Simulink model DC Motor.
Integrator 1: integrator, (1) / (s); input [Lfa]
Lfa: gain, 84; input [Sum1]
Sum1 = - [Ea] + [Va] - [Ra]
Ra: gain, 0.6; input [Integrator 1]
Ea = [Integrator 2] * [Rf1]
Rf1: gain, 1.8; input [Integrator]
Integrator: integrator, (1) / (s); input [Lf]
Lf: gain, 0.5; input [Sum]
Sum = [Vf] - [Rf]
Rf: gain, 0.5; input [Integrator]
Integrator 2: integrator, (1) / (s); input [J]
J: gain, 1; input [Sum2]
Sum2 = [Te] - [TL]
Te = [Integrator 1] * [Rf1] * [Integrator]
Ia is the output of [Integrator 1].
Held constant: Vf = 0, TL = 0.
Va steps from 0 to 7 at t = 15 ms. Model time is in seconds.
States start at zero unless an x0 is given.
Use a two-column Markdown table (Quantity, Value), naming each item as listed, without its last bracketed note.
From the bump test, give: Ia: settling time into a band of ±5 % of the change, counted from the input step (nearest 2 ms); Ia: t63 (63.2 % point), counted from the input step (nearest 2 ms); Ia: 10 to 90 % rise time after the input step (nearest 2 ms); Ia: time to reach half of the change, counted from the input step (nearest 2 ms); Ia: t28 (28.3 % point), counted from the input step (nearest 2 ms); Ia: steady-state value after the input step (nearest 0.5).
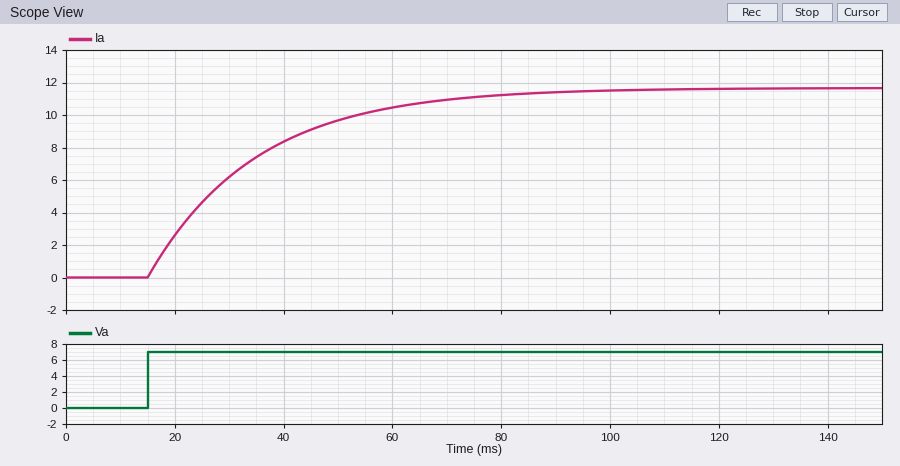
| Quantity | Value |
|---|---|
| Ia: settling time into a band of ±5 % of the change, counted from the input step | 60 ms |
| Ia: t63 (63.2 % point), counted from the input step | 20 ms |
| Ia: 10 to 90 % rise time after the input step | 44 ms |
| Ia: time to reach half of the change, counted from the input step | 14 ms |
| Ia: t28 (28.3 % point), counted from the input step | 6 ms |
| Ia: steady-state value after the input step | 11.5 |
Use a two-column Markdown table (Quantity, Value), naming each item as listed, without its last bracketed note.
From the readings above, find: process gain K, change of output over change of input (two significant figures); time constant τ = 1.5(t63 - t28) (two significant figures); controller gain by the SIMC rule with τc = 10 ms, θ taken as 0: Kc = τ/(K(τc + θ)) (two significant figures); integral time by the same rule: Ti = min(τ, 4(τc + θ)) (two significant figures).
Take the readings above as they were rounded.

| Quantity | Value |
|---|---|
| process gain K, change of output over change of input | 1.6 |
| time constant τ = 1.5(t63 - t28) | 21 ms |
| controller gain by the SIMC rule with τc = 10 ms, θ taken as 0: Kc = τ/(K(τc + θ)) | 1.3 |
| integral time by the same rule: Ti = min(τ, 4(τc + θ)) | 21 ms |
